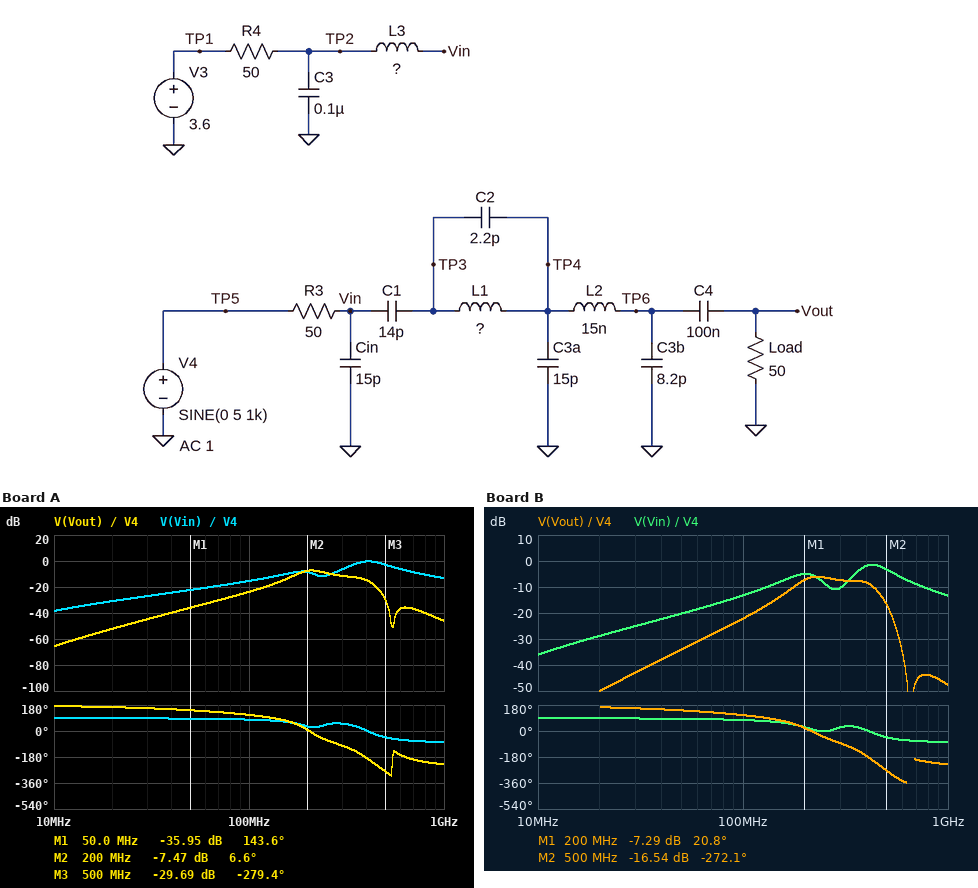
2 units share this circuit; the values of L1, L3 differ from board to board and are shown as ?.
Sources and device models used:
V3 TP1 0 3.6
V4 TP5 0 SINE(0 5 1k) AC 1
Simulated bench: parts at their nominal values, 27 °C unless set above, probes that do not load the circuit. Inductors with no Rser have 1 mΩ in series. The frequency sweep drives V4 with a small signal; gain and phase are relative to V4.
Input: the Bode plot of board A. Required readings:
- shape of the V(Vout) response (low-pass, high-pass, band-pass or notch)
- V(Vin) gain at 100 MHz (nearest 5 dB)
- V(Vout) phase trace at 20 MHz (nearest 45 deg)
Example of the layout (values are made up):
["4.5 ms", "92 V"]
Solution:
["band-pass", "-15 dB", "180 deg"]
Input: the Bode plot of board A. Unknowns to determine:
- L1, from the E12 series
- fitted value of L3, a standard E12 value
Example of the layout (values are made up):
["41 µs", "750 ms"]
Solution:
["39 nH", "12 nH"]
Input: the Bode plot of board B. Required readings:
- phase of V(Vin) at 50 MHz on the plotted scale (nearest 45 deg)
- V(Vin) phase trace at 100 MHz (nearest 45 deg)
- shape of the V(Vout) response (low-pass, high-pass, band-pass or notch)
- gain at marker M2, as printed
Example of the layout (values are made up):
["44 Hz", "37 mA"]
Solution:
["90 deg", "90 deg", "band-pass", "-16.54 dB"]
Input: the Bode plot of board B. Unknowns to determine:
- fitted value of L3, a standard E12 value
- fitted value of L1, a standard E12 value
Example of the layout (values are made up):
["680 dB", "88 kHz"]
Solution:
["15 nH", "27 nH"]
